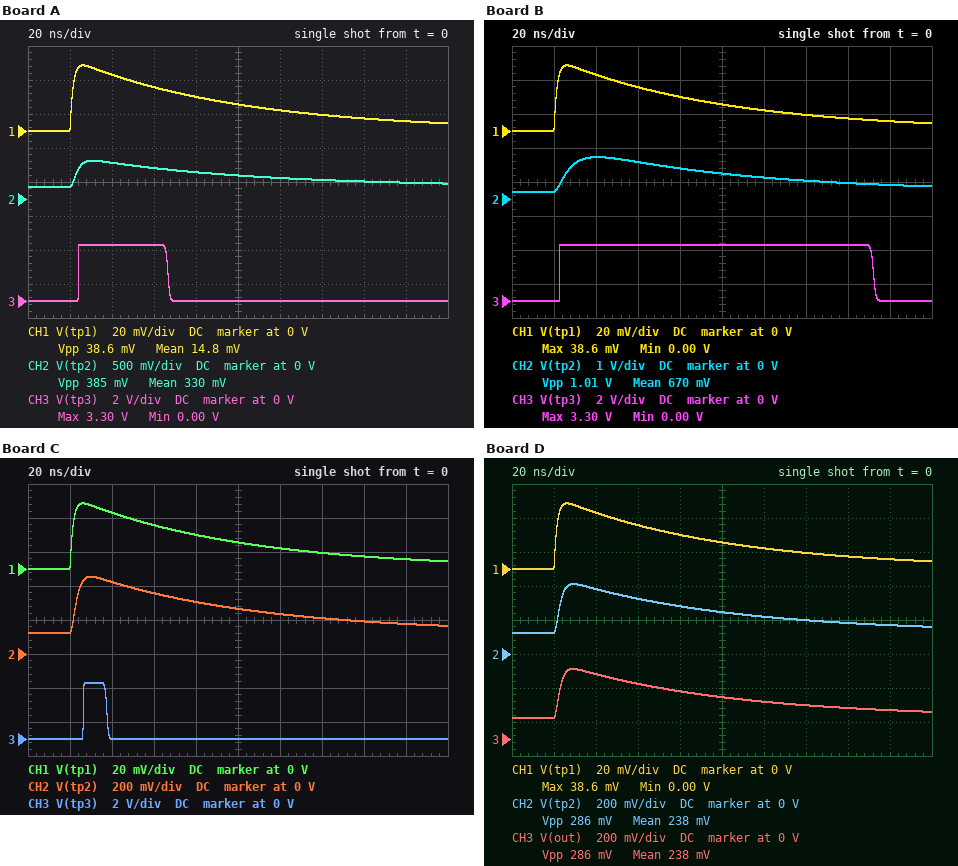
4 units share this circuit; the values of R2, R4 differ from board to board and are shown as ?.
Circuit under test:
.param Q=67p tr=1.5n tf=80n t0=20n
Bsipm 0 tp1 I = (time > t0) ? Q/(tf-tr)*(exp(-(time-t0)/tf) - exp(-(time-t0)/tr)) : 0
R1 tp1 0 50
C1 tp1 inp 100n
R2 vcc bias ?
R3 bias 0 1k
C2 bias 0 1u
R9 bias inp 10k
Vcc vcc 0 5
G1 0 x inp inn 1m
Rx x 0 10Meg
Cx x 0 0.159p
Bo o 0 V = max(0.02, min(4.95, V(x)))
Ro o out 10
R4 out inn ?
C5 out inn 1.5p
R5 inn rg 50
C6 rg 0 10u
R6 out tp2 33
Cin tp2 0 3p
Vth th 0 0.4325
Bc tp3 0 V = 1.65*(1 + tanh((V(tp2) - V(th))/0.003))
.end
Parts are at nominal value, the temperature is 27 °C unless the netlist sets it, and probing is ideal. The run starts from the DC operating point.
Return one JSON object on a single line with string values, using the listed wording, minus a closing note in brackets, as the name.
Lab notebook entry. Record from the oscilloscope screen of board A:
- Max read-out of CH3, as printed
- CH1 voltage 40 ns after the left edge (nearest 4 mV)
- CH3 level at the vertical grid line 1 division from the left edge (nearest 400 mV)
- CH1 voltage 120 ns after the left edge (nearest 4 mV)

{"Max read-out of CH3, as printed": "3.30 V", "CH1 voltage 40 ns after the left edge": "32 mV", "CH3 level at the vertical grid line 1 division from the left edge": "0 V", "CH1 voltage 120 ns after the left edge": "12 mV"}
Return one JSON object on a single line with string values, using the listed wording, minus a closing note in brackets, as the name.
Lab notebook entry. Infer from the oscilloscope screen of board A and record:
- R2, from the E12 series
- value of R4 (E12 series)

{"R2, from the E12 series": "27 kΩ", "value of R4": "470 Ω"}
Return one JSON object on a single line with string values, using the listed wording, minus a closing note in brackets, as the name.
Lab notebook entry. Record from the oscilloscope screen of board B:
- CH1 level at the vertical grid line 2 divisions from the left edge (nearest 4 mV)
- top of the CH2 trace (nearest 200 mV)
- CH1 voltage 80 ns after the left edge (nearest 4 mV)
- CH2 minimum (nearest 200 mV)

{"CH1 level at the vertical grid line 2 divisions from the left edge": "32 mV", "top of the CH2 trace": "1.2 V", "CH1 voltage 80 ns after the left edge": "20 mV", "CH2 minimum": "200 mV"}
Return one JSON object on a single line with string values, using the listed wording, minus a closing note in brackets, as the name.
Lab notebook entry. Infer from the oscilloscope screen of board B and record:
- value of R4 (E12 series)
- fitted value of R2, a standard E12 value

{"value of R4": "1.5 kΩ", "fitted value of R2, a standard E12 value": "22 kΩ"}
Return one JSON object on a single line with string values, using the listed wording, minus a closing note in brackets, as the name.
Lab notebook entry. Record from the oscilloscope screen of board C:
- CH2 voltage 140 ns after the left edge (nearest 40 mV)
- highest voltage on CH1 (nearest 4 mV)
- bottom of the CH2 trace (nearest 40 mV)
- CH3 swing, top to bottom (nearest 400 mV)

{"CH2 voltage 140 ns after the left edge": "200 mV", "highest voltage on CH1": "40 mV", "bottom of the CH2 trace": "120 mV", "CH3 swing, top to bottom": "3.2 V"}
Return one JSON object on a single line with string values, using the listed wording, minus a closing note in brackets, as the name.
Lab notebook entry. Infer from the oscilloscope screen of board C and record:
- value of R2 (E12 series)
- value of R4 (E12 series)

{"value of R2": "39 kΩ", "value of R4": "390 Ω"}
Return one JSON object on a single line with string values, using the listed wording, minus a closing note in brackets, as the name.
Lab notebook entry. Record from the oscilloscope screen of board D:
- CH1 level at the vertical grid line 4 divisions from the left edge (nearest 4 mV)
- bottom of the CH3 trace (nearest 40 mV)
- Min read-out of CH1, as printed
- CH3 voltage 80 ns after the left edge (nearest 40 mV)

{"CH1 level at the vertical grid line 4 divisions from the left edge": "20 mV", "bottom of the CH3 trace": "120 mV", "Min read-out of CH1, as printed": "0.00 V", "CH3 voltage 80 ns after the left edge": "280 mV"}
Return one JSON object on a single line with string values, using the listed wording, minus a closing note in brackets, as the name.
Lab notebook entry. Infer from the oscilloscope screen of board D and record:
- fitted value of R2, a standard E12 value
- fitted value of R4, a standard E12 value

{"fitted value of R2, a standard E12 value": "39 kΩ", "fitted value of R4, a standard E12 value": "330 Ω"}
